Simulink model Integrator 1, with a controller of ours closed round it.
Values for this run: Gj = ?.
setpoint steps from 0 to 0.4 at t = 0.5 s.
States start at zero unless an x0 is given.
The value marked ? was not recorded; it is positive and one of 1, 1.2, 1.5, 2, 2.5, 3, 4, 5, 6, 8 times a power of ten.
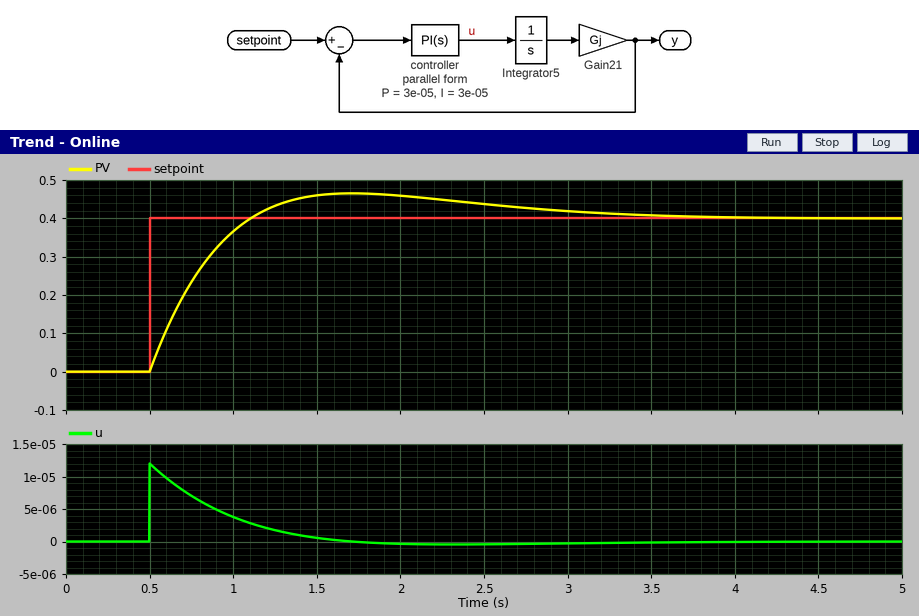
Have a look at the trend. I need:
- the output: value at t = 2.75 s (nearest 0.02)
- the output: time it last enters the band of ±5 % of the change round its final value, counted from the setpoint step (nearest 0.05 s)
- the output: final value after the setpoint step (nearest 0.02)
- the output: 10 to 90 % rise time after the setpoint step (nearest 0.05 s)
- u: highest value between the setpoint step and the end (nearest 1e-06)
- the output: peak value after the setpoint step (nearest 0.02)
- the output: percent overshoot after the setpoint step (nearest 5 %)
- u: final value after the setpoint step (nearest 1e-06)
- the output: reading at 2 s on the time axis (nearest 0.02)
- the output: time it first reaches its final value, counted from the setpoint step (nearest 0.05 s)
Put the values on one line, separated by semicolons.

0.42; 2.45 s; 0.40; 0.45 s; 0.000012; 0.46; 15 %; 0.000000; 0.46; 0.60 s
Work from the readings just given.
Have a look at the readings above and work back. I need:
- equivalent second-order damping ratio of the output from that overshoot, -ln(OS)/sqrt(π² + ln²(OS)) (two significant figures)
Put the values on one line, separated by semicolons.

0.52
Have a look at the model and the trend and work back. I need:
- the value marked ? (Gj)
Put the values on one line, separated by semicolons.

100000
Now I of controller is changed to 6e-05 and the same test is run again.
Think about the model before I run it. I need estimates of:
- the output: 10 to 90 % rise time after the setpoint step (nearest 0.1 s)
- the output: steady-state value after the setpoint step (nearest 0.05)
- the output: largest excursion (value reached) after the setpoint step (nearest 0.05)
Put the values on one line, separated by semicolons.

0.4 s; 0.40; 0.50
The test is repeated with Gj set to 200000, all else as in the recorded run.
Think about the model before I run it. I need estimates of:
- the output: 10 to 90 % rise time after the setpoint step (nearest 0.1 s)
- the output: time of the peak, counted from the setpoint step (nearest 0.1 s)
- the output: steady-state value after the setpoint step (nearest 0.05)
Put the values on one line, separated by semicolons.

0.3 s; 0.8 s; 0.40
